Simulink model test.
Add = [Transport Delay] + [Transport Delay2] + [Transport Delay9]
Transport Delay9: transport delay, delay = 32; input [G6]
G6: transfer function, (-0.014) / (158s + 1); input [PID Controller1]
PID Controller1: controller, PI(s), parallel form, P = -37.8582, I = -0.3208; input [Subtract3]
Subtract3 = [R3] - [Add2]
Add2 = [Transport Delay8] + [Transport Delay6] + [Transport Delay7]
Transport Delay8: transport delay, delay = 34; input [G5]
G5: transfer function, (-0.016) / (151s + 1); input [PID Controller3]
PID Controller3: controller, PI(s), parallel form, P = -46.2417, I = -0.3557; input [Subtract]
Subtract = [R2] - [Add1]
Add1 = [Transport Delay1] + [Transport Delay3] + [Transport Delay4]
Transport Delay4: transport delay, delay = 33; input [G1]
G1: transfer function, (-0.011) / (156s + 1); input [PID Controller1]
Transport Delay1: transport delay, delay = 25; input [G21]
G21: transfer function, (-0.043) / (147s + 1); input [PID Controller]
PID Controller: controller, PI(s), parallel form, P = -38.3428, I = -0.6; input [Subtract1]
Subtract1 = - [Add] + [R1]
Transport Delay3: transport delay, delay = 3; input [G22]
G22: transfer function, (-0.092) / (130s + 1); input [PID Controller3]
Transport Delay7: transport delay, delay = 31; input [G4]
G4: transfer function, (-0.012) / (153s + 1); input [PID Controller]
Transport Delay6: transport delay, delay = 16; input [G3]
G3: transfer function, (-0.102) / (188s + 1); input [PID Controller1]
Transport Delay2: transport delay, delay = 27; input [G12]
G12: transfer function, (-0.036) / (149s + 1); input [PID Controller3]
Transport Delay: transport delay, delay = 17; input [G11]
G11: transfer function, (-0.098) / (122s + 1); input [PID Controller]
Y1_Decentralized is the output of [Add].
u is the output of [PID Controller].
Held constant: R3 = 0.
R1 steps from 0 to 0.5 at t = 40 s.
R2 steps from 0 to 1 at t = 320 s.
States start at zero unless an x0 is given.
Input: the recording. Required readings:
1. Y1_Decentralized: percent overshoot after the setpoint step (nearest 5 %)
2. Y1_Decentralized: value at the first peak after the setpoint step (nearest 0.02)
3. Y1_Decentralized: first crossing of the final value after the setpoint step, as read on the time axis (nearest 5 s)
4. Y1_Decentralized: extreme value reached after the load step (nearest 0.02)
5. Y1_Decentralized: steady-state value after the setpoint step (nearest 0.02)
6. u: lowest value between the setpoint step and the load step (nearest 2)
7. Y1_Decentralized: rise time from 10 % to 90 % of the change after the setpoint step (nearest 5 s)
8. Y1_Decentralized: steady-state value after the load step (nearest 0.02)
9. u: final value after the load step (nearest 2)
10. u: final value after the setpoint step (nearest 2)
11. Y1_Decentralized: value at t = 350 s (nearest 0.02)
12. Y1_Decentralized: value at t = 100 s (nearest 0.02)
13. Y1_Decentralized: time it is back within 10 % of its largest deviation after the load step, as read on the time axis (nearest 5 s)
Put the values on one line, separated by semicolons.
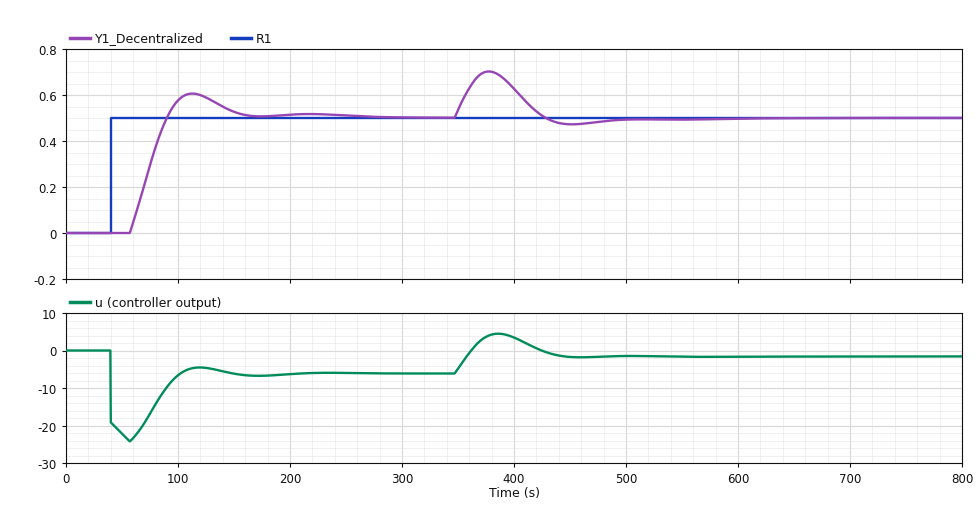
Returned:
20 %; 0.60; 90 s; 0.70; 0.50; -24; 25 s; 0.50; -2; -6; 0.54; 0.58; 470 s
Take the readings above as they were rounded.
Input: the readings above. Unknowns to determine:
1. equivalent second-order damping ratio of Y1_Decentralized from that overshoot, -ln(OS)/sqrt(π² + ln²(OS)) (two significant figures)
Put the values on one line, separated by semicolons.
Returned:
0.46
